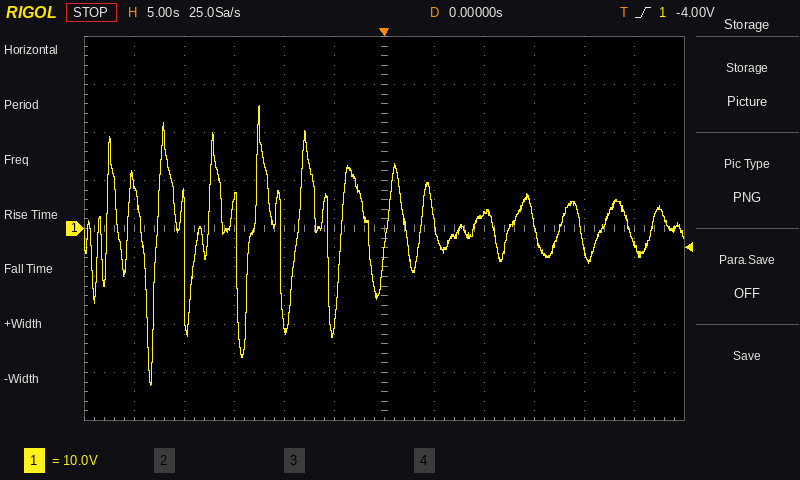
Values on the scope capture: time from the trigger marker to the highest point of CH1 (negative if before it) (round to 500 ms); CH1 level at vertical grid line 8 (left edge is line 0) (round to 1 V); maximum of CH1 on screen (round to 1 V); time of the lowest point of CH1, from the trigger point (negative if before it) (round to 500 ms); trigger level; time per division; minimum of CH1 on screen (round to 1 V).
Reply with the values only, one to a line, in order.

-12.5 s
3 V
26 V
-23.5 s
-4.00 V
5 s
-33 V
